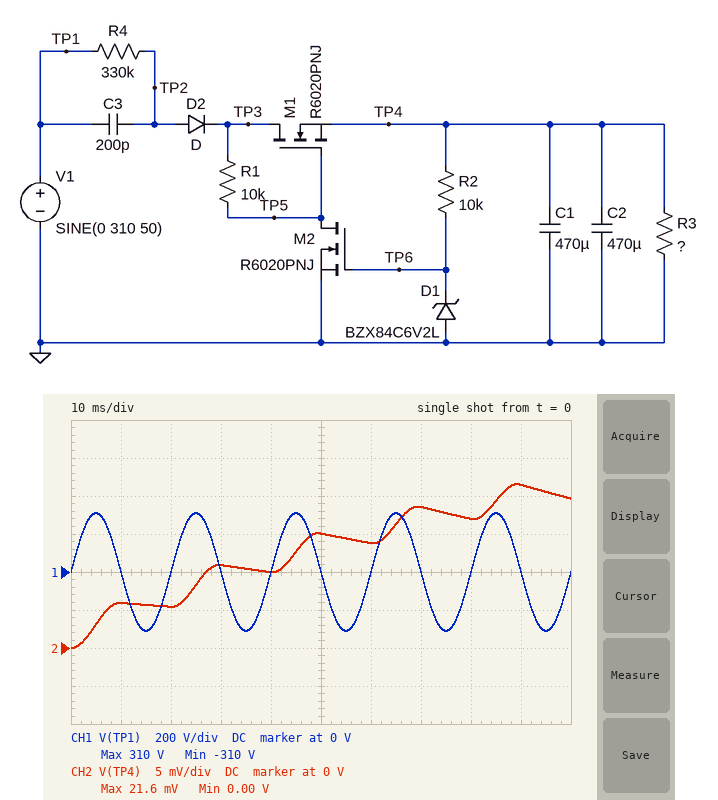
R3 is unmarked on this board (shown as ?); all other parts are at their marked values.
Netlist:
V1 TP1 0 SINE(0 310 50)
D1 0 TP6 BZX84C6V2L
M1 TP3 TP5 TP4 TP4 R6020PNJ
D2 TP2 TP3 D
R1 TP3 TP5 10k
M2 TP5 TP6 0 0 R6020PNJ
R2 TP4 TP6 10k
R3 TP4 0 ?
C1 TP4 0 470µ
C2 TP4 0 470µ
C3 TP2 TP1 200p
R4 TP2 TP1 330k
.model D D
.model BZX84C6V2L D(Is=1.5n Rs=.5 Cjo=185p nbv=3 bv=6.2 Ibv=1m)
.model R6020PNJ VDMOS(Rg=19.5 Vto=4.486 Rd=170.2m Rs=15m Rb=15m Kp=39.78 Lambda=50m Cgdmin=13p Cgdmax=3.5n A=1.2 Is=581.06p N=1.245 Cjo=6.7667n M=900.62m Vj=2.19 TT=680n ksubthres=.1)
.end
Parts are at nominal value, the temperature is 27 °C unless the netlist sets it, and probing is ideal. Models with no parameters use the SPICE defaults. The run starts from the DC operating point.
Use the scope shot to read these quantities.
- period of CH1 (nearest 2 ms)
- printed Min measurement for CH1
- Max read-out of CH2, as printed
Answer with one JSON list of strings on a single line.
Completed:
["20 ms", "-310 V", "21.6 mV"]
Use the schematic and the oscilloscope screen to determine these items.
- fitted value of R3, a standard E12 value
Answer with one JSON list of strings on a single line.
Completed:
["120 Ω"]
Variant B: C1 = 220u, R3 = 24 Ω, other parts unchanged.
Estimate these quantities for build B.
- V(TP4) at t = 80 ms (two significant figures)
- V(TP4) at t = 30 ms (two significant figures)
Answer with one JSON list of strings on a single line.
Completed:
["4.9 mV", "8.2 mV"]
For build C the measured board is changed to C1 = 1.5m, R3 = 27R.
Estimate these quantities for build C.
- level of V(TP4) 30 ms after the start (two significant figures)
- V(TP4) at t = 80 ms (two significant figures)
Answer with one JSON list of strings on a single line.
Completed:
["4.5 mV", "5.5 mV"]
